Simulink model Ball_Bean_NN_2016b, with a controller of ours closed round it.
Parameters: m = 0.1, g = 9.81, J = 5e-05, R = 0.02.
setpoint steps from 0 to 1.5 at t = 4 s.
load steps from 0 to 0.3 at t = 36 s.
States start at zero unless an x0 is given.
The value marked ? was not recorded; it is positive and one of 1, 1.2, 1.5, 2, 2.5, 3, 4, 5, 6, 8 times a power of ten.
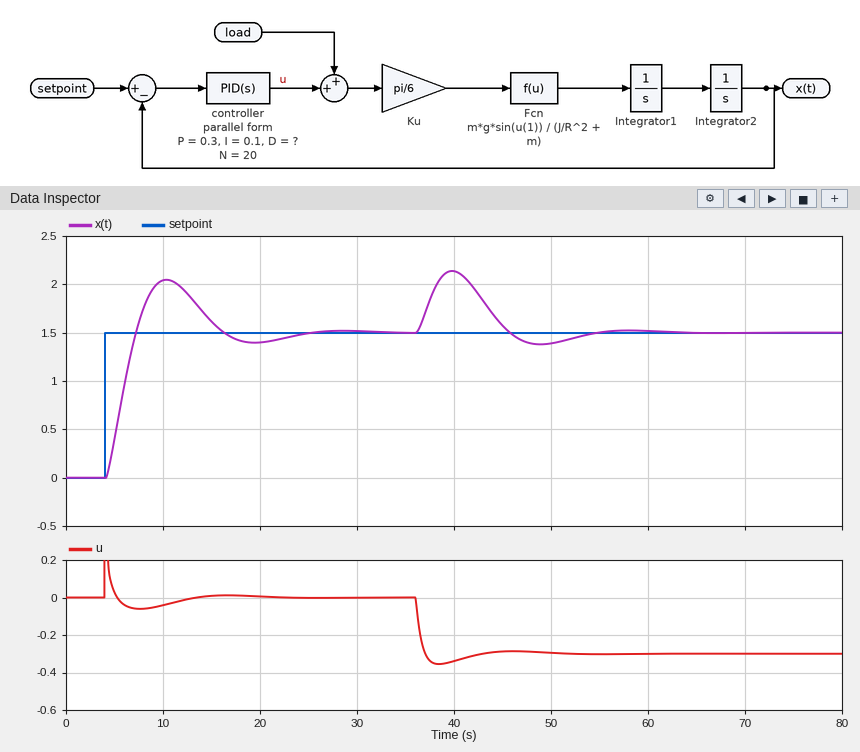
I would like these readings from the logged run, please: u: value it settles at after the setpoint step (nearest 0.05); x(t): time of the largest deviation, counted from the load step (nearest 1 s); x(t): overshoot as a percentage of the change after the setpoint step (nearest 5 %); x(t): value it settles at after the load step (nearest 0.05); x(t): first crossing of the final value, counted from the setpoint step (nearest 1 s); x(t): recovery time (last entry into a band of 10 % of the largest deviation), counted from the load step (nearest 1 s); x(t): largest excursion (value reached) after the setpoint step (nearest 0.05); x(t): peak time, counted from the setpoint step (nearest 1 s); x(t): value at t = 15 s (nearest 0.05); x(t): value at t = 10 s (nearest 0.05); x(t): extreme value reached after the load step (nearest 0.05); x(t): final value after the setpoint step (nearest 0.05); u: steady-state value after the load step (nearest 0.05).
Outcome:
0.00
4 s
35 %
1.50
3 s
16 s
2.05
6 s
1.60
2.05
2.15
1.50
-0.30
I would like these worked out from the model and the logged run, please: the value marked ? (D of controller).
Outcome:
0.8
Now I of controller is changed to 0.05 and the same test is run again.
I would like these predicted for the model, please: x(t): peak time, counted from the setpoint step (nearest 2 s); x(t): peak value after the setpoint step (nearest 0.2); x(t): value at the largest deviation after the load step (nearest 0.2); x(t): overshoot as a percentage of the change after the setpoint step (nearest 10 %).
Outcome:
8 s
1.8
2.2
20 %
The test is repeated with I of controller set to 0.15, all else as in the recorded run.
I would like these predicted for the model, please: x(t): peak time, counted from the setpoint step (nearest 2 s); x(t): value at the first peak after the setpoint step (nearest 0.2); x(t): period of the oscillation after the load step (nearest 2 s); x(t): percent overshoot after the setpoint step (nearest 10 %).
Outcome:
6 s
2.2
14 s
50 %
